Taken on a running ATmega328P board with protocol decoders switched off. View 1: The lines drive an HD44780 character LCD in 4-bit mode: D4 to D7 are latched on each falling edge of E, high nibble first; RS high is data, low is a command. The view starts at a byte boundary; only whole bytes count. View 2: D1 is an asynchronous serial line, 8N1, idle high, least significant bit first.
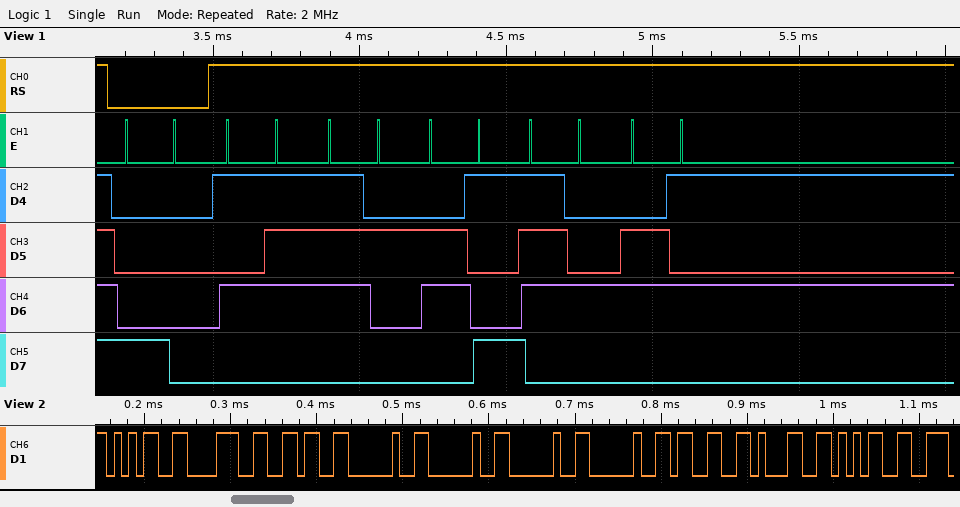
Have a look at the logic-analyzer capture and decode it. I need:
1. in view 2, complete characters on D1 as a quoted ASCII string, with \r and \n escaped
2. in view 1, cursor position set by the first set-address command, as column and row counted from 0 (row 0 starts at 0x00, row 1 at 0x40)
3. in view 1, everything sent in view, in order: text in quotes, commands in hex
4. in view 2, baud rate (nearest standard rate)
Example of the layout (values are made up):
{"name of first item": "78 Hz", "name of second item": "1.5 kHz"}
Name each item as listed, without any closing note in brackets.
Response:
{"in view 2, complete characters on D1 as a quoted ASCII string, with \\r and \\n escaped": "\"586    315\"", "in view 1, cursor position set by the first set-address command, as column and row counted from 0": "column 0, row 0", "in view 1, everything sent in view, in order: text in quotes, commands in hex": "0x80 \"Write\"", "in view 2, baud rate": "115200 baud"}
